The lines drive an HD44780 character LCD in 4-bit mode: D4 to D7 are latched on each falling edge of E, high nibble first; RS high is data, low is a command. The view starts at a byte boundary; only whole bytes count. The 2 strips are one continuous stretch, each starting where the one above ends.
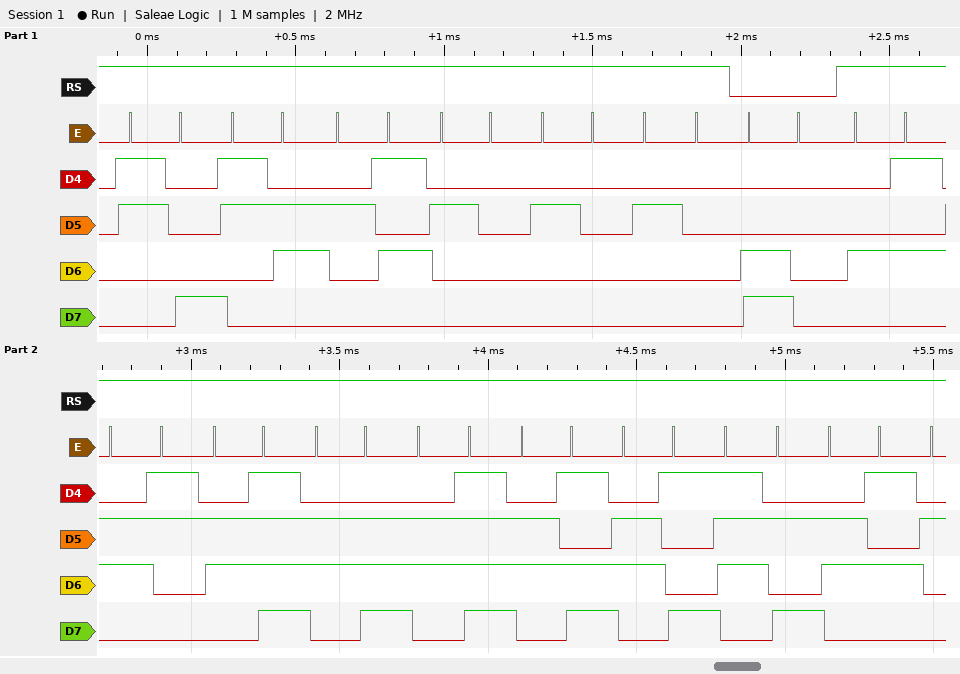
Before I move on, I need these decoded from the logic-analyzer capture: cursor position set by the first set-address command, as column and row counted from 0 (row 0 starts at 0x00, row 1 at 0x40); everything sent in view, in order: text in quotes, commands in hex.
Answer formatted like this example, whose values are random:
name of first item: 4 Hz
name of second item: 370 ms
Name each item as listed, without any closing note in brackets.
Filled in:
cursor position set by the first set-address command, as column and row counted from 0: column 0, row 1
everything sent in view, in order: text in quotes, commands in hex: "86%   " 0xC0 "Economize"
